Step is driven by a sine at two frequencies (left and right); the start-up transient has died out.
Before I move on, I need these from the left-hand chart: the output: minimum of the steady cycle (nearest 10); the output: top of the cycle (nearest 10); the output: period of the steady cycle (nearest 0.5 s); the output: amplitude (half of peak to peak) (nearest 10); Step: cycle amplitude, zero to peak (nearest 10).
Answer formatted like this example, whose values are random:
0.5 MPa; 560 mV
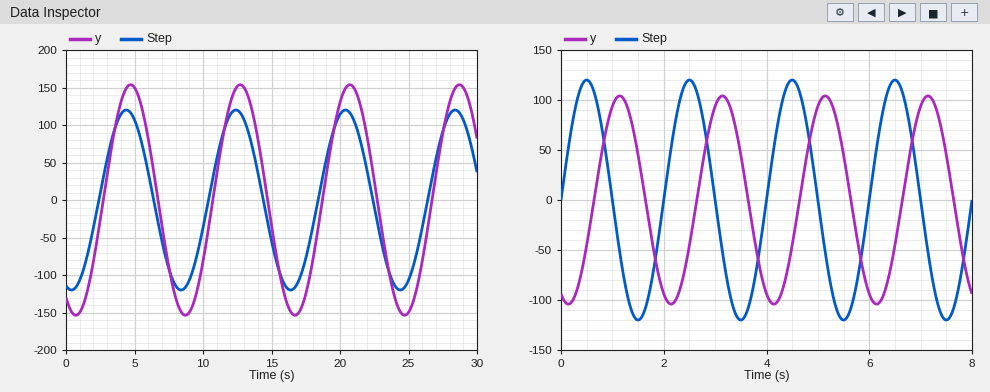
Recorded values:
-150; 150; 8.0 s; 150; 120
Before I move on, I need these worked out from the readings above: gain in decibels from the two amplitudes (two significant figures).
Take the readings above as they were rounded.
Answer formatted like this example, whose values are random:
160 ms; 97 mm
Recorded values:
1.9 dB
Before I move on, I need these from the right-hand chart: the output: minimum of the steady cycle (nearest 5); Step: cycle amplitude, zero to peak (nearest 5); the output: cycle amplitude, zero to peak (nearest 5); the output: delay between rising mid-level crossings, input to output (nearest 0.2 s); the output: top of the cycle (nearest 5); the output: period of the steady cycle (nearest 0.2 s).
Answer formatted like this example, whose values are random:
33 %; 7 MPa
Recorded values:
-105; 120; 105; 0.6 s; 105; 2.0 s
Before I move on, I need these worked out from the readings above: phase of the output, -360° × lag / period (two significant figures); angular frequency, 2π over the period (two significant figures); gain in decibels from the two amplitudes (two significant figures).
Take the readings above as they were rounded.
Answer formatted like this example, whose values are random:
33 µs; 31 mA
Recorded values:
-110°; 3.1 rad/s; -1.2 dB
